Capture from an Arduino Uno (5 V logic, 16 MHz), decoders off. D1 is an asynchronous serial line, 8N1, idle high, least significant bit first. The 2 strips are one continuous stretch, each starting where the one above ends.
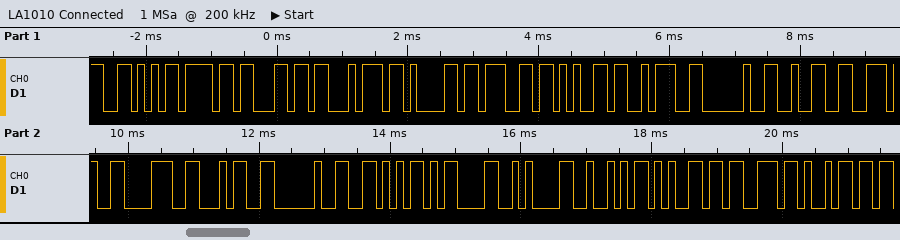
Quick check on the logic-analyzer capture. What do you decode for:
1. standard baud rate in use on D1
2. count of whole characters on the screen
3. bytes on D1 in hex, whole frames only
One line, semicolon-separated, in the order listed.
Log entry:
9600 baud; 21; 56 6F 6C 74 61 67 65 3A 20 32 2E 38 34 20 56 0D 0A 52 65 73 69
